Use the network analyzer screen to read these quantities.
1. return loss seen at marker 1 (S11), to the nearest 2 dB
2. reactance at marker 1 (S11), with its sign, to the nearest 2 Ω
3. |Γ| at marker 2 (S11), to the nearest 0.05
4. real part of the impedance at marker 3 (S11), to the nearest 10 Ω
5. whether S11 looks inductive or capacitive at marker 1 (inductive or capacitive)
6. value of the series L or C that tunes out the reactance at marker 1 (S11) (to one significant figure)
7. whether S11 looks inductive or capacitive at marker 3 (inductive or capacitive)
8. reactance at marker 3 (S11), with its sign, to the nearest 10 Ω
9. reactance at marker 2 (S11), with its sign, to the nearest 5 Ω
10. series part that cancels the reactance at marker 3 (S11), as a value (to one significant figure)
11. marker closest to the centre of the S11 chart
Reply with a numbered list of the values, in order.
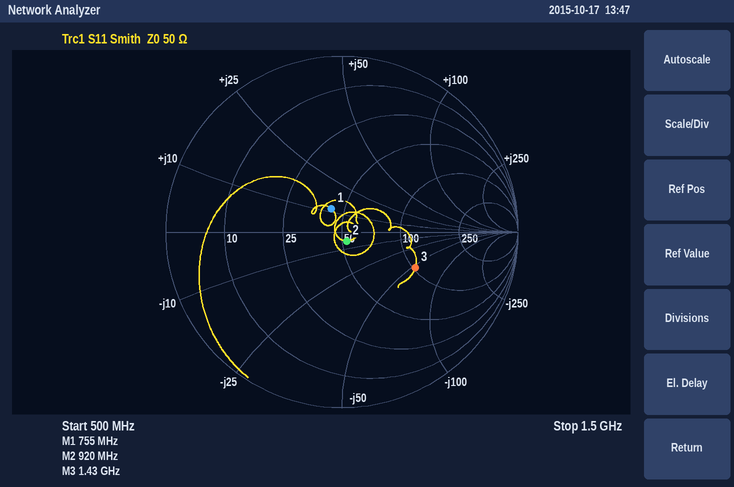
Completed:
1. 16 dB
2. +12 Ω
3. 0.05
4. 100 Ω
5. inductive
6. 20 pF
7. capacitive
8. -50 Ω
9. -5 Ω
10. 6 nH
11. marker 2
